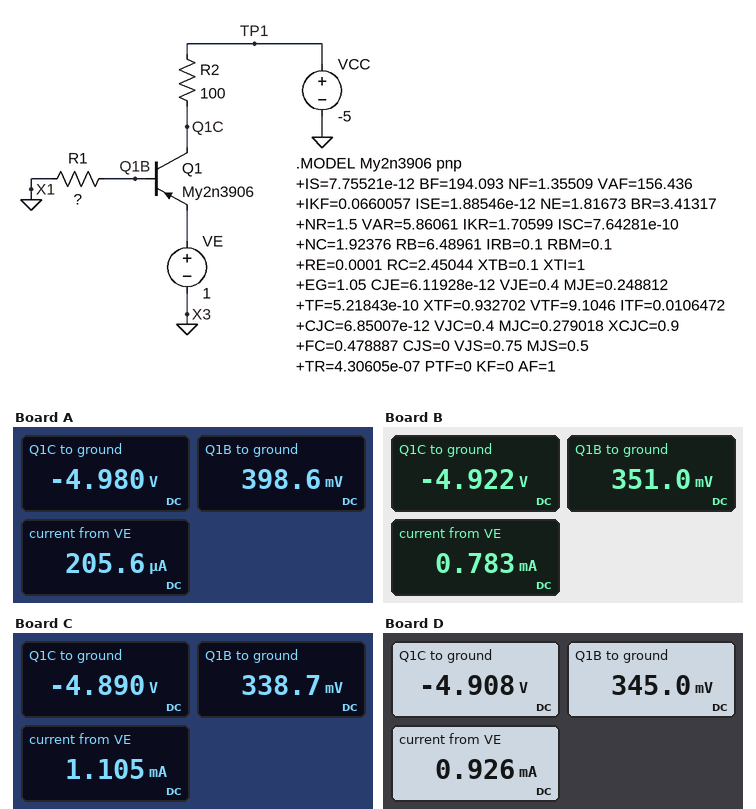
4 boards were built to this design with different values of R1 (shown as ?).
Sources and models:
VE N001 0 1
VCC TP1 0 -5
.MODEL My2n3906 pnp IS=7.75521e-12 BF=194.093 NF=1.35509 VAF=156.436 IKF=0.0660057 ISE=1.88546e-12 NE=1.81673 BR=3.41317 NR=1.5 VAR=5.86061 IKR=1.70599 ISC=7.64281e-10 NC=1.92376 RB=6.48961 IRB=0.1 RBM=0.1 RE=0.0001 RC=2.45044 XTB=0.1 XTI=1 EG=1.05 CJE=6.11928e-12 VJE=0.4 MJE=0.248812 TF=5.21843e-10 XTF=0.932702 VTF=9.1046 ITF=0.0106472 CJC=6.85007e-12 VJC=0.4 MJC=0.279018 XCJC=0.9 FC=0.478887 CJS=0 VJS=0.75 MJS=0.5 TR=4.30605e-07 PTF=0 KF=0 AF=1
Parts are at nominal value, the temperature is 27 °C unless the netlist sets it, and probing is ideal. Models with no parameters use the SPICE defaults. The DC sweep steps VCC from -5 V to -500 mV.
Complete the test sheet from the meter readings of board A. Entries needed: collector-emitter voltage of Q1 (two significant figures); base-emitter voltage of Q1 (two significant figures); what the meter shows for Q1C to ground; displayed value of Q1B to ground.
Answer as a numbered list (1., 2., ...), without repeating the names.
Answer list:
1. -6.0 V
2. -600 mV
3. -4.980 V
4. 398.6 mV
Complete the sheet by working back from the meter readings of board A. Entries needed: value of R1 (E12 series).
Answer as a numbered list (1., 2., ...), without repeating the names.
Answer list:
1. 220 kΩ
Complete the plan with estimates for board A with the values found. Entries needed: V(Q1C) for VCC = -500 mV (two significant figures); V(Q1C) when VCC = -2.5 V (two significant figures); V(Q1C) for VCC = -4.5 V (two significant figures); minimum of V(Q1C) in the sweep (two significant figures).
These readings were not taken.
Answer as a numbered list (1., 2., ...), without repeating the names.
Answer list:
1. -480 mV
2. -2.5 V
3. -4.5 V
4. -5.0 V
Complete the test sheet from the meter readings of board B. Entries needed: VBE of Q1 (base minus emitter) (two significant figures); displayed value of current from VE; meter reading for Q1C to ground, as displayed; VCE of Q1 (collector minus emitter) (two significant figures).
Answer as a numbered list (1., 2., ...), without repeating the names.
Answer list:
1. -650 mV
2. 0.783 mA
3. -4.922 V
4. -5.9 V
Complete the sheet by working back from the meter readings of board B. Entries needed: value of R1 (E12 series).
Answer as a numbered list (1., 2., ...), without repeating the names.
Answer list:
1. 56 kΩ
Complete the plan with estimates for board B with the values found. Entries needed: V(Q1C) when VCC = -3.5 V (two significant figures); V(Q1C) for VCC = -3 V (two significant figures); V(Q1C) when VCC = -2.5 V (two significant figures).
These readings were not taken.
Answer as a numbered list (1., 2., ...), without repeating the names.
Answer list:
1. -3.4 V
2. -2.9 V
3. -2.4 V
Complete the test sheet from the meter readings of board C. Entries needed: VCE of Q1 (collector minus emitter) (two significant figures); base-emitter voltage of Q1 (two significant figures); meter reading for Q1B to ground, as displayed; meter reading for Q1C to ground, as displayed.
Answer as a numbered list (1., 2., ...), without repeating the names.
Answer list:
1. -5.9 V
2. -660 mV
3. 338.7 mV
4. -4.890 V
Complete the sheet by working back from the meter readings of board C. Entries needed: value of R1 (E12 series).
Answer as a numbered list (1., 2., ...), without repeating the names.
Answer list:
1. 39 kΩ
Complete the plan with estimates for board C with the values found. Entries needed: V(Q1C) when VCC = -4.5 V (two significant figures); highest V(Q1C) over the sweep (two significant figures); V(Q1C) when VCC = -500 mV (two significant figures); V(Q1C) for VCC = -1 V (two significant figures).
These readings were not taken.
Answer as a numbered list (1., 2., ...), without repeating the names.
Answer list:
1. -4.4 V
2. -390 mV
3. -390 mV
4. -890 mV
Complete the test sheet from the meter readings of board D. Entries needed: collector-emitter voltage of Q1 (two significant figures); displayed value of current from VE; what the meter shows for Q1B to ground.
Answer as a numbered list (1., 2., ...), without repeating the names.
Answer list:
1. -5.9 V
2. 0.926 mA
3. 345.0 mV
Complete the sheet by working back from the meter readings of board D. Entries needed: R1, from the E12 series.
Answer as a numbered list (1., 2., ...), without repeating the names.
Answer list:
1. 47 kΩ
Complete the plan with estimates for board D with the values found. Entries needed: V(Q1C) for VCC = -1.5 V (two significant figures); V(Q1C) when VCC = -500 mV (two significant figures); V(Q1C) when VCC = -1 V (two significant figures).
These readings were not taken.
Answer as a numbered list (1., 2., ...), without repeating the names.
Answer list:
1. -1.4 V
2. -410 mV
3. -910 mV
